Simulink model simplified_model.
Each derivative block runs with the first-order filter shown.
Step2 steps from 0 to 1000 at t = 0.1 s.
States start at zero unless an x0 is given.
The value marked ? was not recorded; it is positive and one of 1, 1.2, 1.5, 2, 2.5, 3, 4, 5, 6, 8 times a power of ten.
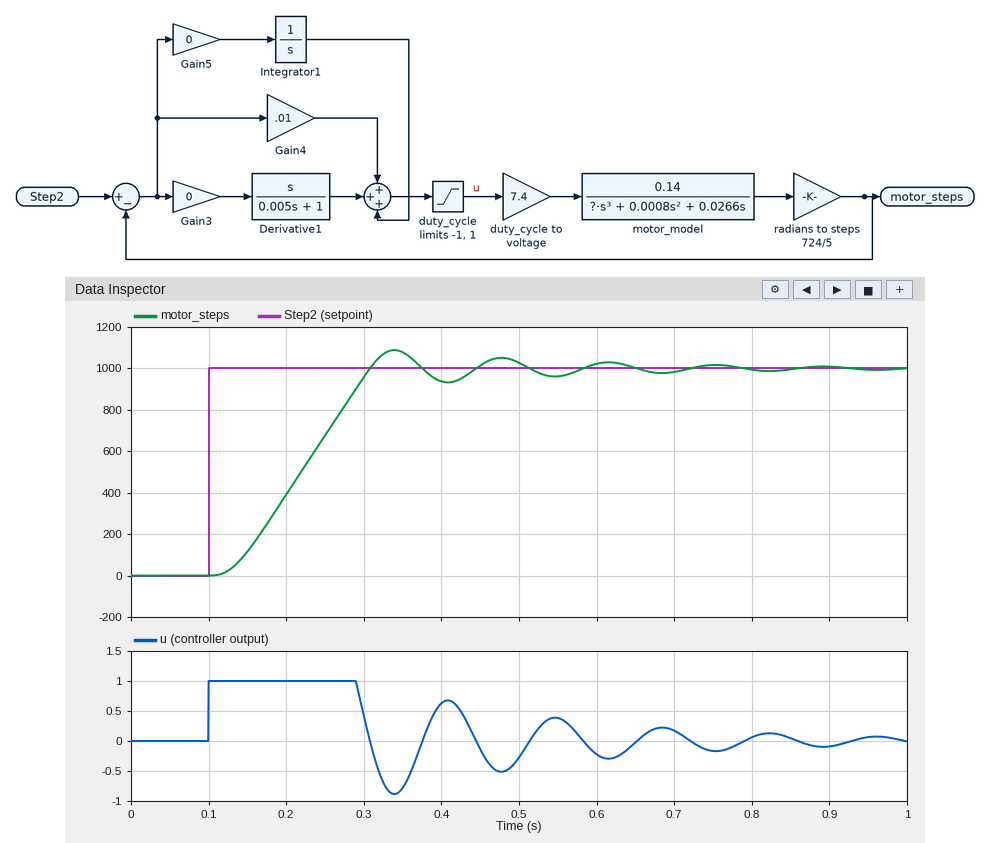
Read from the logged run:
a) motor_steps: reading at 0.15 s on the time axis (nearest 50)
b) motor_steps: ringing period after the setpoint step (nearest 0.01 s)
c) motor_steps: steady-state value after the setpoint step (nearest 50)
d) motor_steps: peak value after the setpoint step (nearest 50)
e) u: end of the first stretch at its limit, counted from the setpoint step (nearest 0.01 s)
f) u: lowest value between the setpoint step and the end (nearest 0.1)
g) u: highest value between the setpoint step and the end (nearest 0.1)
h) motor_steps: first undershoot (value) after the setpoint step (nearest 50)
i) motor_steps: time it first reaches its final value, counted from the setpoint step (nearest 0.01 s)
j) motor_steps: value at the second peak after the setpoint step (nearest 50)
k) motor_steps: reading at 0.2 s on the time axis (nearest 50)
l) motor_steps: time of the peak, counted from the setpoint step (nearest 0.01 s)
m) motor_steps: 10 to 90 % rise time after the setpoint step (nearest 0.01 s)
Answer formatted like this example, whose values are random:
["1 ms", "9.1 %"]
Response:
["100", "0.14 s", "1000", "1100", "0.19 s", "-0.9", "1.0", "950", "0.21 s", "1050", "400", "0.24 s", "0.14 s"]
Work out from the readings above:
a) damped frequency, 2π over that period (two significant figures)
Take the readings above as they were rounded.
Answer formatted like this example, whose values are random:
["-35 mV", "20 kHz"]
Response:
["45 rad/s"]
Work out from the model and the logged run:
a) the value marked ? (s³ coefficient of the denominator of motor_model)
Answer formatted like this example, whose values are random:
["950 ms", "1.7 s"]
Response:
["1e-05"]
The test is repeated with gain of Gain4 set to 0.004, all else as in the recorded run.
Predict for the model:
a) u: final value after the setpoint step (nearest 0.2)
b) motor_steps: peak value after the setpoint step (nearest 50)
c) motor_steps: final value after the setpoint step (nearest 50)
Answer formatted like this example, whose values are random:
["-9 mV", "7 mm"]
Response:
["0.0", "1050", "1000"]
